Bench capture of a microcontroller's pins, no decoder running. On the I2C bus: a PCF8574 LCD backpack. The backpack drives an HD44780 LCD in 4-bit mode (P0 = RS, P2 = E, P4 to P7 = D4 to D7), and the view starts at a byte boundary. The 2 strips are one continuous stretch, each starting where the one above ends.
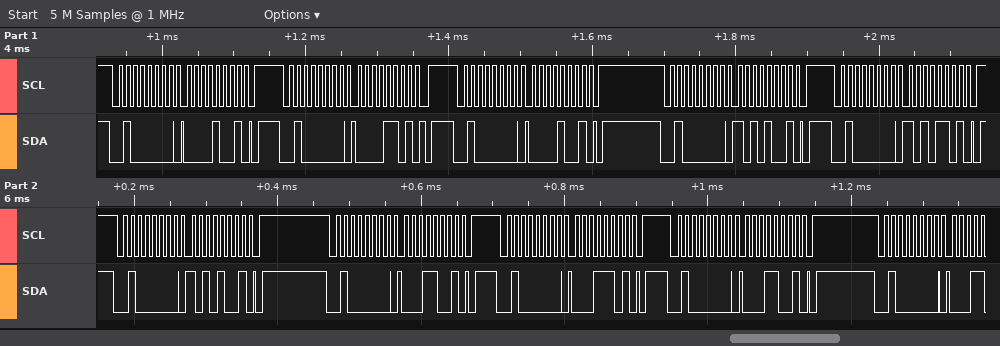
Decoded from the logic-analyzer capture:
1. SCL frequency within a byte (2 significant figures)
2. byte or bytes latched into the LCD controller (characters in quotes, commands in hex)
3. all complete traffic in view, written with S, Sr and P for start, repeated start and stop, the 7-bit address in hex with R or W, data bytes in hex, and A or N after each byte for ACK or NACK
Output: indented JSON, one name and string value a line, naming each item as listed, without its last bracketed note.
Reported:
{
  "SCL frequency within a byte": "100 kHz",
  "byte or bytes latched into the LCD controller": "data 0x0A",
  "all complete traffic in view, written with S, Sr and P for start, repeated start and stop, the 7-bit address in hex with R or W, data bytes in hex, and A or N after each byte for ACK or NACK": "S 20W A 09 A P S 20W A 0D A P S 20W A 09 A P S 20W A A9 A P S 20W A AD A P S 20W A A9 A P S 20W A 19 A P S 20W A 1D A P S 20W A 19 A P S 20W A"
}
